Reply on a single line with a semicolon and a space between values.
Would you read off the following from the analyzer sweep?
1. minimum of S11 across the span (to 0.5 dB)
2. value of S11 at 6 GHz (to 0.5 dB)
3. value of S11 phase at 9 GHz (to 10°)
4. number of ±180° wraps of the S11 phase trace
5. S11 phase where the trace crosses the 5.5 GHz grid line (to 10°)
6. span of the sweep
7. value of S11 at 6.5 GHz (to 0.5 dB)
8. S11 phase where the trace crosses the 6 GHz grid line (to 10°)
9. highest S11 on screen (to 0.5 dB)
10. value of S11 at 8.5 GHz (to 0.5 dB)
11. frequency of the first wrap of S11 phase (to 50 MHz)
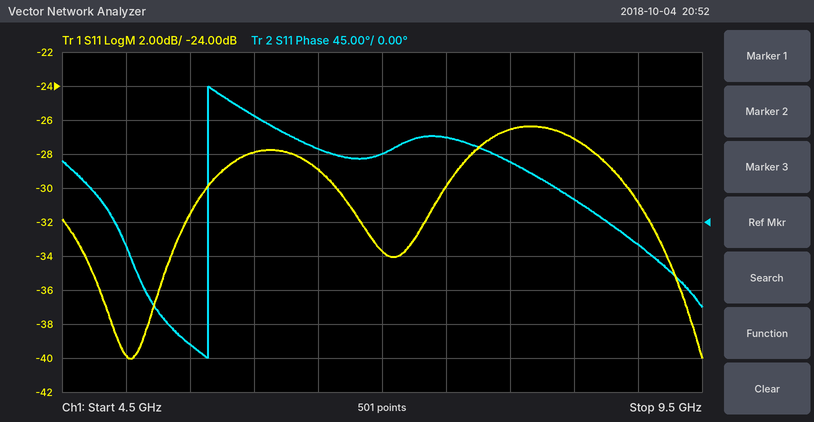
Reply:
-40.0 dB; -28.0 dB; -30°; 1; -160°; 5 GHz; -29.0 dB; 140°; -26.5 dB; -27.0 dB; 5.65 GHz
